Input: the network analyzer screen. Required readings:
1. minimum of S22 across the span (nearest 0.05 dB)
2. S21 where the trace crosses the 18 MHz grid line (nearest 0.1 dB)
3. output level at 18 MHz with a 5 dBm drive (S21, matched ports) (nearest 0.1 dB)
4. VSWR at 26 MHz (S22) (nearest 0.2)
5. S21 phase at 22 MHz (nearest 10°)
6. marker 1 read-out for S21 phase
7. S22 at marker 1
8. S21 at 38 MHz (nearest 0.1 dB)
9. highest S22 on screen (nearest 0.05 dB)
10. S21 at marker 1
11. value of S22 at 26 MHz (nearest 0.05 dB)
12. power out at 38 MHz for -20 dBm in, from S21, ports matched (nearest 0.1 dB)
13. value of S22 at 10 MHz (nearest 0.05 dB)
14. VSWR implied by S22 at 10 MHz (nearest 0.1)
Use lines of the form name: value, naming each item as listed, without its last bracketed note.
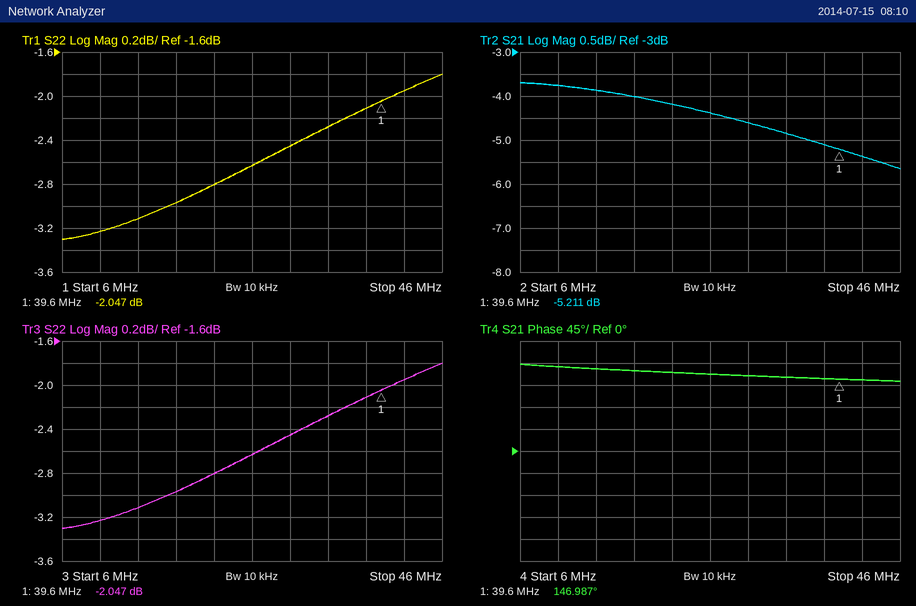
minimum of S22 across the span: -3.30 dB
S21 where the trace crosses the 18 MHz grid line: -4.0 dB
output level at 18 MHz with a 5 dBm drive (S21, matched ports): 1.0 dBm
VSWR at 26 MHz (S22): 6.6
S21 phase at 22 MHz: 160°
marker 1 read-out for S21 phase: 146.987°
S22 at marker 1: -2.047 dB
S21 at 38 MHz: -5.1 dB
highest S22 on screen: -1.80 dB
S21 at marker 1: -5.211 dB
value of S22 at 26 MHz: -2.65 dB
power out at 38 MHz for -20 dBm in, from S21, ports matched: -25.1 dBm
value of S22 at 10 MHz: -3.25 dB
VSWR implied by S22 at 10 MHz: 5.4
